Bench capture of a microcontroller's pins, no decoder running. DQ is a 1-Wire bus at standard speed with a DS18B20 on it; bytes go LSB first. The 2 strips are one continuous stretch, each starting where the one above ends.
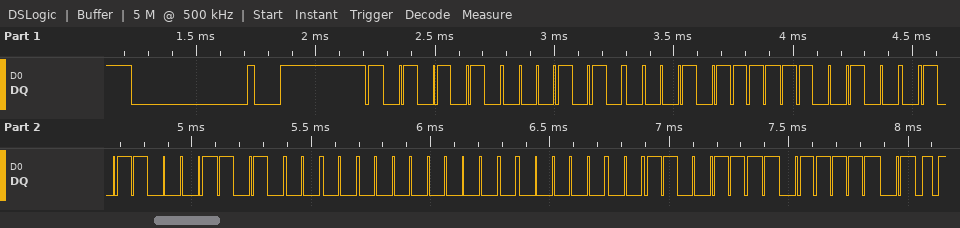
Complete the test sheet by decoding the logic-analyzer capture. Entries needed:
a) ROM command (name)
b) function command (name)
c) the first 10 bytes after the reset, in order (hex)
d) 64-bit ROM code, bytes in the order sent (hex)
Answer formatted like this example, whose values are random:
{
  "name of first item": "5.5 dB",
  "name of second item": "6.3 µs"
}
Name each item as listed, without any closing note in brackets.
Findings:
{
  "ROM command": "Match ROM",
  "function command": "Read Scratchpad",
  "the first 10 bytes after the reset, in order": "55 28 F4 13 8D 05 00 00 F3 BE",
  "64-bit ROM code, bytes in the order sent": "28 F4 13 8D 05 00 00 F3"
}
